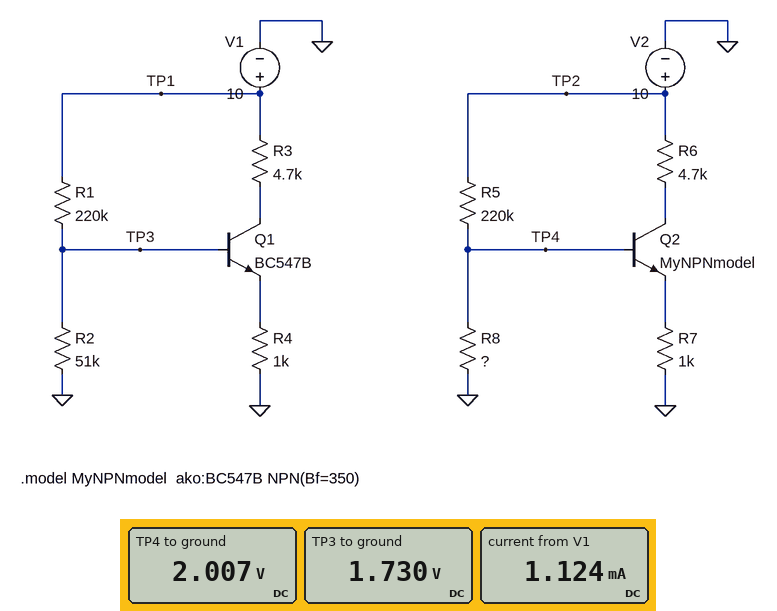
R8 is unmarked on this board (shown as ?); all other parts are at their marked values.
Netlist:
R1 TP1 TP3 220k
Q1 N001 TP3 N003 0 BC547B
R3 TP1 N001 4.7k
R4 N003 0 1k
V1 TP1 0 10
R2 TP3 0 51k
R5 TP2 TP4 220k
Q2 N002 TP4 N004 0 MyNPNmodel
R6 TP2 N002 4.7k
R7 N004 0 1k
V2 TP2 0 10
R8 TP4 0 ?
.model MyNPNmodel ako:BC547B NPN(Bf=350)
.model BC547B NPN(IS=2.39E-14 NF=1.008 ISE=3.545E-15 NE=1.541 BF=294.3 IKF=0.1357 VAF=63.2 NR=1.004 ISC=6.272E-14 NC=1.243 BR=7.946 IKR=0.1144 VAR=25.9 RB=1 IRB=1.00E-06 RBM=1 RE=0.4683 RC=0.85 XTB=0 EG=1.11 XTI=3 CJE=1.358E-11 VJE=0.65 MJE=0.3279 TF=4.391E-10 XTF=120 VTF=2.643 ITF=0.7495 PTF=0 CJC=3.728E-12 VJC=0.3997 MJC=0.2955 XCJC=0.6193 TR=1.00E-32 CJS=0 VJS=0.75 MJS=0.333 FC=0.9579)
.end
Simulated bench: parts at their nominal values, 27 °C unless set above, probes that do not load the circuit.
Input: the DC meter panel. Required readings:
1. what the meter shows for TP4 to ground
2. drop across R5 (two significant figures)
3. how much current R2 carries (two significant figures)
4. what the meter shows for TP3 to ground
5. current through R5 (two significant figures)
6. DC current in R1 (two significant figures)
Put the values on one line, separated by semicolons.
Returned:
2.007 V; 8.0 V; 34 µA; 1.730 V; 36 µA; 38 µA
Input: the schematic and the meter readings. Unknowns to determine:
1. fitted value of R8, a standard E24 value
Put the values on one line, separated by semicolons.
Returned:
62 kΩ
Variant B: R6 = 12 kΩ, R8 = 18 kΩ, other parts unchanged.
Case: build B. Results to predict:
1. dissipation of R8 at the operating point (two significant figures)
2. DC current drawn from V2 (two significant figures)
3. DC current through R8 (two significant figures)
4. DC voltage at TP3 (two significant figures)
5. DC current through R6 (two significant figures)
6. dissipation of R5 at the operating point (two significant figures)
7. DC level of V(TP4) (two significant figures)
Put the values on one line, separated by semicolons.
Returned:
31 µW; 200 µA; 42 µA; 1.7 V; 160 µA; 390 µW; 750 mV
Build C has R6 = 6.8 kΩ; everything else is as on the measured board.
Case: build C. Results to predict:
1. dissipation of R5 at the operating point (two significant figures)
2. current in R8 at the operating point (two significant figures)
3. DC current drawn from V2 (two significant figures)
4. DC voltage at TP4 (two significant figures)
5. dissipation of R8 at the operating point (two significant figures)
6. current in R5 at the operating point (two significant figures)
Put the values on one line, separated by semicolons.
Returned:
300 µW; 31 µA; 1.3 mA; 1.9 V; 59 µW; 37 µA
